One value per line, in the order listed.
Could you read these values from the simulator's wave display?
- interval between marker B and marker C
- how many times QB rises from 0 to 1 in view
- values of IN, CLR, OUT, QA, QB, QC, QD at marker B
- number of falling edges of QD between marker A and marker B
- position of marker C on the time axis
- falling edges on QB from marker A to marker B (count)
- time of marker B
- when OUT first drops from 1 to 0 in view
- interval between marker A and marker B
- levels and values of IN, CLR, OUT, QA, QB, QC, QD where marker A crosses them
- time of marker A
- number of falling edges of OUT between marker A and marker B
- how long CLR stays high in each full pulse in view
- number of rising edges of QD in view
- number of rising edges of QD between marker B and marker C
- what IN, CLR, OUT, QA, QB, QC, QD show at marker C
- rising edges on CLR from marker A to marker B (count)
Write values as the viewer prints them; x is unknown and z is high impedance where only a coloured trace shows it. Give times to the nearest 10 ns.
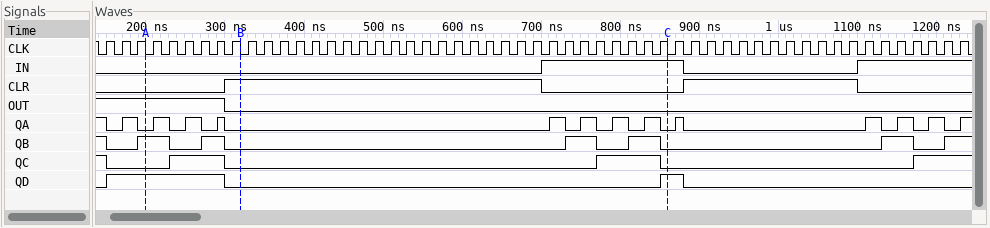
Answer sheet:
540 ns
6
IN=0, CLR=1, OUT=0, QA=0, QB=0, QC=0, QD=0
1
860 ns
2
320 ns
300 ns
120 ns
IN=0, CLR=0, OUT=1, QA=0, QB=1, QC=0, QD=1
200 ns
1
400 ns, 220 ns
2
1
IN=1, CLR=0, OUT=0, QA=0, QB=0, QC=0, QD=1
1
